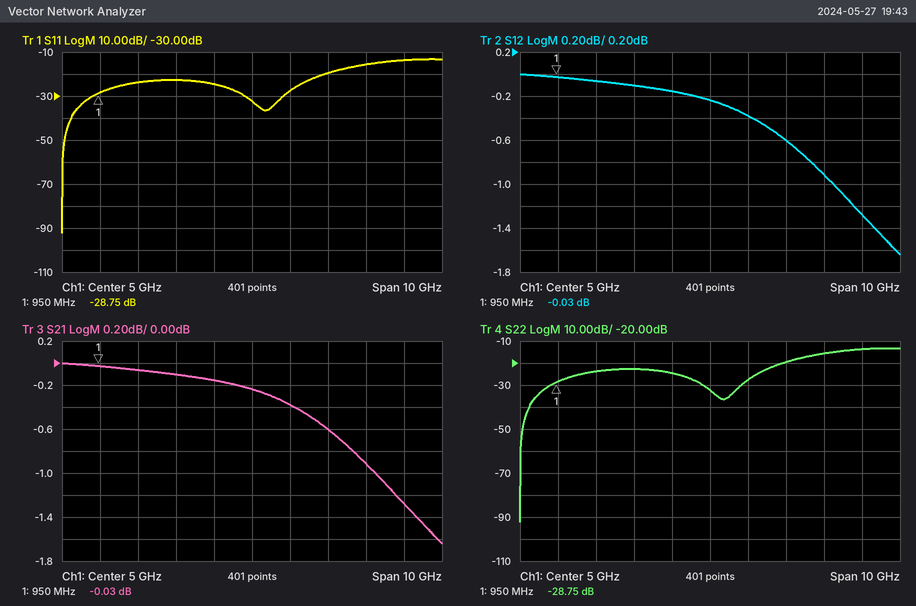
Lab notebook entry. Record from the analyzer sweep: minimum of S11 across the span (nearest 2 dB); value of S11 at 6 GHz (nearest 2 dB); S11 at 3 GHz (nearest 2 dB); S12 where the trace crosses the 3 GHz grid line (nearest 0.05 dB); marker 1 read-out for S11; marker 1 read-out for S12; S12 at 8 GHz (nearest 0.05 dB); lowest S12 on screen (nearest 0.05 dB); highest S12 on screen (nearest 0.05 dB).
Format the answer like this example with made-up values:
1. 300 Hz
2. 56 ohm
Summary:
1. -92 dB
2. -28 dB
3. -22 dB
4. -0.10 dB
5. -28.75 dB
6. -0.03 dB
7. -0.90 dB
8. -1.65 dB
9. 0.00 dB
